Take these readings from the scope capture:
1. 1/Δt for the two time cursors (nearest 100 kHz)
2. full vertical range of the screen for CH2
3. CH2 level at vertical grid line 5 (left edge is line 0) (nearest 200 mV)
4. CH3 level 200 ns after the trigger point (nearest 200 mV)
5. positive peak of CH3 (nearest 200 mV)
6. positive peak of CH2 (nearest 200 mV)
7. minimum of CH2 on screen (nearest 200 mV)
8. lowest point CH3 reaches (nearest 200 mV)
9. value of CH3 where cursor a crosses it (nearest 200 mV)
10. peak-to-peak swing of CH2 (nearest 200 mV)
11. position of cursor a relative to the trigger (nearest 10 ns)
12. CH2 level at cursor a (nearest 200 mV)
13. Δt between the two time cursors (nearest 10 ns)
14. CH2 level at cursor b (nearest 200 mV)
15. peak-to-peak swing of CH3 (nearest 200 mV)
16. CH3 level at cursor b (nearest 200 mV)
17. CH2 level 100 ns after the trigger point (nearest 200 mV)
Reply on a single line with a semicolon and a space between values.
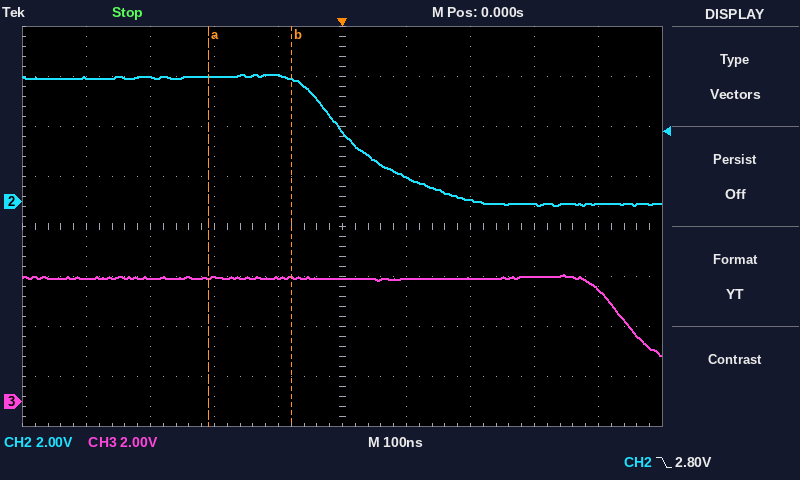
7.7 MHz; 16 V; 2.8 V; 5.0 V; 5.0 V; 5.0 V; -200 mV; 1.8 V; 5.0 V; 5.2 V; -210 ns; 5.0 V; 130 ns; 4.8 V; 3.2 V; 5.0 V; 1.0 V
